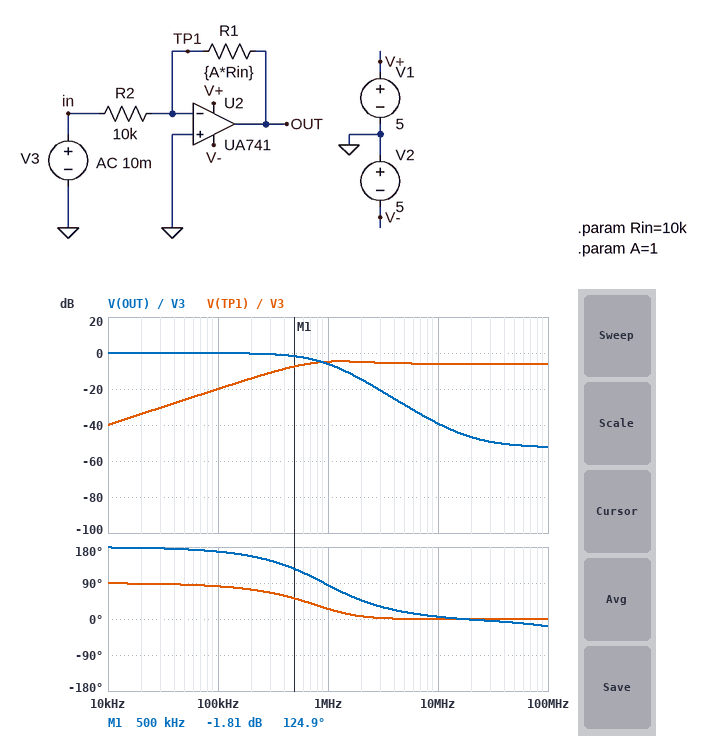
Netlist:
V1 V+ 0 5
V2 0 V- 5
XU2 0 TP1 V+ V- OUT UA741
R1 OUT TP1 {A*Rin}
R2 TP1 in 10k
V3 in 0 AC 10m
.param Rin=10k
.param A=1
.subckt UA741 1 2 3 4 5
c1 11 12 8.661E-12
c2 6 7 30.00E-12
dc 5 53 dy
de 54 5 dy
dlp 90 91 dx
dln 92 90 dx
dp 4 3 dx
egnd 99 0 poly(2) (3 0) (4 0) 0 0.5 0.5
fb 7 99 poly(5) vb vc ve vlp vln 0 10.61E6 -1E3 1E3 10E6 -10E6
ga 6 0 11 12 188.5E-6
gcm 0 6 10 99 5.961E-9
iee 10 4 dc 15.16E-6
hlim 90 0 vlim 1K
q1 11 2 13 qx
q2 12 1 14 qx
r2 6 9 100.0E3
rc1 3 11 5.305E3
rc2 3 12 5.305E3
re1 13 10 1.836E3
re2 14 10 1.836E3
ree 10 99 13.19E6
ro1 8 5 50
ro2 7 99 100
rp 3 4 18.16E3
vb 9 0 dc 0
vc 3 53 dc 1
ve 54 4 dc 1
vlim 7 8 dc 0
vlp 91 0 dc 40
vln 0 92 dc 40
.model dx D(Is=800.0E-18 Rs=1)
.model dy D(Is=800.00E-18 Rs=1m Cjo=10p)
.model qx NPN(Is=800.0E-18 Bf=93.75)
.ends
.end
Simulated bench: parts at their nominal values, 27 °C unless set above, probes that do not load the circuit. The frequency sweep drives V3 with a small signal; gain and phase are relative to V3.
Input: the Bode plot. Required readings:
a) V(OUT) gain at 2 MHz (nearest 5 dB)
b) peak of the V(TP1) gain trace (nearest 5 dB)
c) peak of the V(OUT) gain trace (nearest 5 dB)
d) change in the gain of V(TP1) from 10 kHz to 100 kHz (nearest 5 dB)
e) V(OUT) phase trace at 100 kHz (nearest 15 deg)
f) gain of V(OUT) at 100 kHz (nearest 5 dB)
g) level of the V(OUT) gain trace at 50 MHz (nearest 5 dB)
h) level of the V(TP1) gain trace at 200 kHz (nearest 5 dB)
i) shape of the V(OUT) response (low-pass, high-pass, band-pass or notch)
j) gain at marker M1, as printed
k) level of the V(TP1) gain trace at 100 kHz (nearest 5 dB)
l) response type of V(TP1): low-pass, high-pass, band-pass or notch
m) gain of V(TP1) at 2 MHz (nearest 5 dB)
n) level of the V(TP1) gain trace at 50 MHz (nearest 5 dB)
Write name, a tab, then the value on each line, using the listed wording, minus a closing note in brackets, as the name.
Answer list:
V(OUT) gain at 2 MHz	-15 dB
peak of the V(TP1) gain trace	-5 dB
peak of the V(OUT) gain trace	0 dB
change in the gain of V(TP1) from 10 kHz to 100 kHz	20 dB
V(OUT) phase trace at 100 kHz	165 deg
gain of V(OUT) at 100 kHz	0 dB
level of the V(OUT) gain trace at 50 MHz	-50 dB
level of the V(TP1) gain trace at 200 kHz	-15 dB
shape of the V(OUT) response	low-pass
gain at marker M1, as printed	-1.81 dB
level of the V(TP1) gain trace at 100 kHz	-20 dB
response type of V(TP1): low-pass, high-pass, band-pass or notch	high-pass
gain of V(TP1) at 2 MHz	-5 dB
level of the V(TP1) gain trace at 50 MHz	-5 dB
